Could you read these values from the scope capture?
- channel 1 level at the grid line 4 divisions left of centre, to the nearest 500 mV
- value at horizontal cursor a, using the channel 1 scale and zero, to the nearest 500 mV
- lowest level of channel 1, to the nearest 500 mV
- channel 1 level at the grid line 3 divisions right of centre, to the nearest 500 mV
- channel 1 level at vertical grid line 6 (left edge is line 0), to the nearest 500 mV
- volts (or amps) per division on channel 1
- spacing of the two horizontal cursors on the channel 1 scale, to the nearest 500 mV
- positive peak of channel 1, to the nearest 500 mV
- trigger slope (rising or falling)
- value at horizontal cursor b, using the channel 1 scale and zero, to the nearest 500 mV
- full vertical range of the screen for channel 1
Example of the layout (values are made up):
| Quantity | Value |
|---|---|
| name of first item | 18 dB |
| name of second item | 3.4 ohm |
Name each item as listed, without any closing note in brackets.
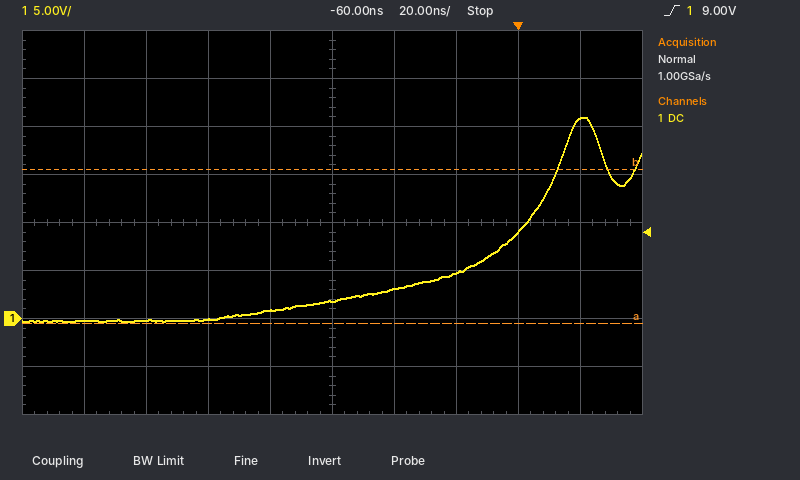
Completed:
| Quantity | Value |
|---|---|
| channel 1 level at the grid line 4 divisions left of centre, to the nearest 500 mV | 0.0 V |
| value at horizontal cursor a, using the channel 1 scale and zero, to the nearest 500 mV | -500 mV |
| lowest level of channel 1, to the nearest 500 mV | -500 mV |
| channel 1 level at the grid line 3 divisions right of centre, to the nearest 500 mV | 9.0 V |
| channel 1 level at vertical grid line 6 (left edge is line 0), to the nearest 500 mV | 3.0 V |
| volts (or amps) per division on channel 1 | 5 V |
| spacing of the two horizontal cursors on the channel 1 scale, to the nearest 500 mV | 16.0 V |
| positive peak of channel 1, to the nearest 500 mV | 21.0 V |
| trigger slope | rising |
| value at horizontal cursor b, using the channel 1 scale and zero, to the nearest 500 mV | 15.5 V |
| full vertical range of the screen for channel 1 | 40 V |
